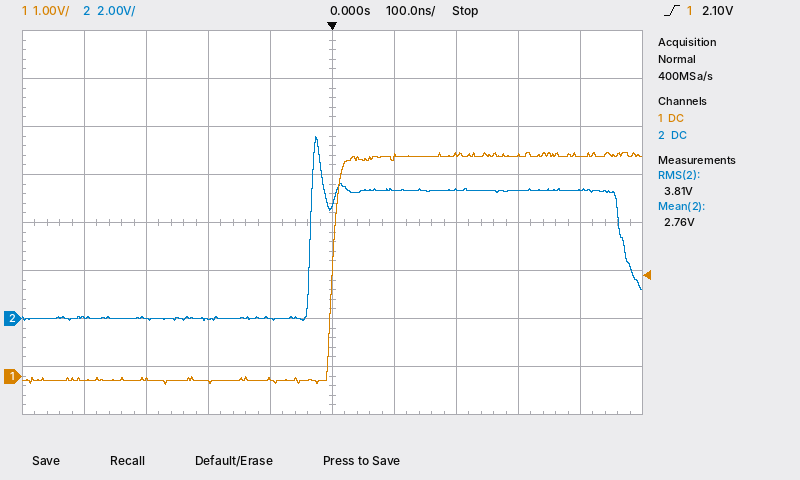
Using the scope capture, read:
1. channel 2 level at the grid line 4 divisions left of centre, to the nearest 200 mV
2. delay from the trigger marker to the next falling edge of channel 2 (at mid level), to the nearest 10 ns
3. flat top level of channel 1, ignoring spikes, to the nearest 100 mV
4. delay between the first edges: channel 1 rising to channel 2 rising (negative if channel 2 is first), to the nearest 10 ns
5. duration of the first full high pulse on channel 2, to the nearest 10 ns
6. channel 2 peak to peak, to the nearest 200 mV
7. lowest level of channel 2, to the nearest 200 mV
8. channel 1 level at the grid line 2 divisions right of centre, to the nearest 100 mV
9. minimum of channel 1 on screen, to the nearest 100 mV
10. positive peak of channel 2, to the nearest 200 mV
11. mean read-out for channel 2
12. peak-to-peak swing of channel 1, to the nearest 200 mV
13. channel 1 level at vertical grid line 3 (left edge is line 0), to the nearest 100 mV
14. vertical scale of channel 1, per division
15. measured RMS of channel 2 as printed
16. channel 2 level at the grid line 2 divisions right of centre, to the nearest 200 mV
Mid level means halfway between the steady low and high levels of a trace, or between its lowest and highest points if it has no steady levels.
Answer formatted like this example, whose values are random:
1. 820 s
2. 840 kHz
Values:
1. 0.0 V
2. 470 ns
3. 4.6 V
4. -40 ns
5. 510 ns
6. 7.6 V
7. 0.0 V
8. 4.6 V
9. -200 mV
10. 7.6 V
11. 2.76 V
12. 4.8 V
13. -100 mV
14. 1 V
15. 3.81 V
16. 5.4 V
